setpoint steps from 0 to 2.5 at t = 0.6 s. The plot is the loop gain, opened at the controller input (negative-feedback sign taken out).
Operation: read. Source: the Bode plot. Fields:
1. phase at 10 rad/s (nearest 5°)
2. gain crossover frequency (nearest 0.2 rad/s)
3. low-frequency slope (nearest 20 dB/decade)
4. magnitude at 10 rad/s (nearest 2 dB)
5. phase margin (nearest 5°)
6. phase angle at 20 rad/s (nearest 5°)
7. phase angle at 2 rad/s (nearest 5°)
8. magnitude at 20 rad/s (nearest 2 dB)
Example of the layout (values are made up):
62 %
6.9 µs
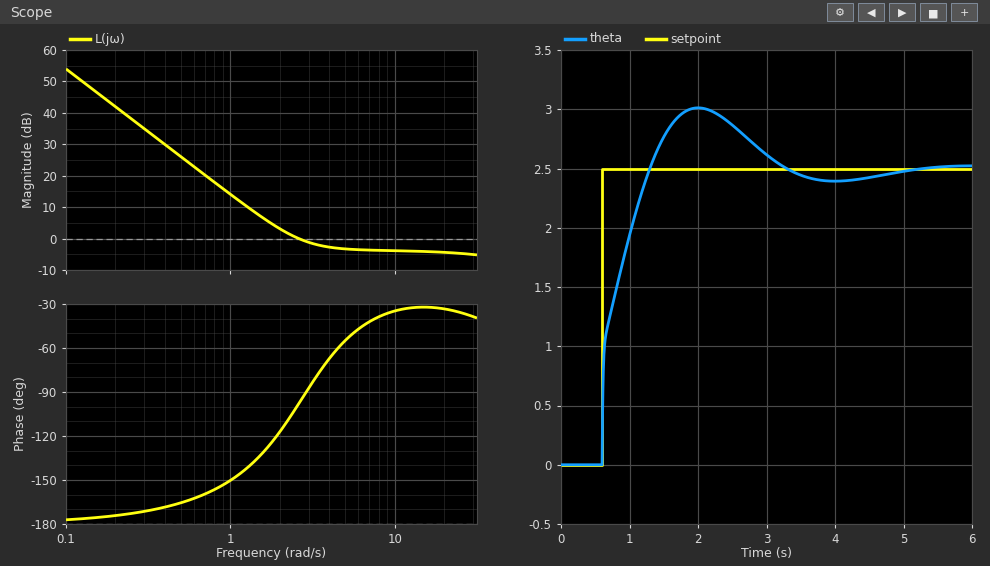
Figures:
-35°
2.6 rad/s
-40 dB/decade
-4 dB
80°
-35°
-115°
-4 dB
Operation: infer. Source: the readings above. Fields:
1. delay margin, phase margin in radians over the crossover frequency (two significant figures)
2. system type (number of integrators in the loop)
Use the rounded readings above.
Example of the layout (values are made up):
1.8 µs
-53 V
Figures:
0.54 s
2
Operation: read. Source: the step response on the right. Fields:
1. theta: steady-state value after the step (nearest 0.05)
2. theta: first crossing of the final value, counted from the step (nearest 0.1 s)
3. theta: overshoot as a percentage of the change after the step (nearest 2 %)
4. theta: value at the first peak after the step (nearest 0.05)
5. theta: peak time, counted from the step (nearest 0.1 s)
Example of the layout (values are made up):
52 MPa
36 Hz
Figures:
2.50
0.7 s
20 %
3.00
1.4 s
